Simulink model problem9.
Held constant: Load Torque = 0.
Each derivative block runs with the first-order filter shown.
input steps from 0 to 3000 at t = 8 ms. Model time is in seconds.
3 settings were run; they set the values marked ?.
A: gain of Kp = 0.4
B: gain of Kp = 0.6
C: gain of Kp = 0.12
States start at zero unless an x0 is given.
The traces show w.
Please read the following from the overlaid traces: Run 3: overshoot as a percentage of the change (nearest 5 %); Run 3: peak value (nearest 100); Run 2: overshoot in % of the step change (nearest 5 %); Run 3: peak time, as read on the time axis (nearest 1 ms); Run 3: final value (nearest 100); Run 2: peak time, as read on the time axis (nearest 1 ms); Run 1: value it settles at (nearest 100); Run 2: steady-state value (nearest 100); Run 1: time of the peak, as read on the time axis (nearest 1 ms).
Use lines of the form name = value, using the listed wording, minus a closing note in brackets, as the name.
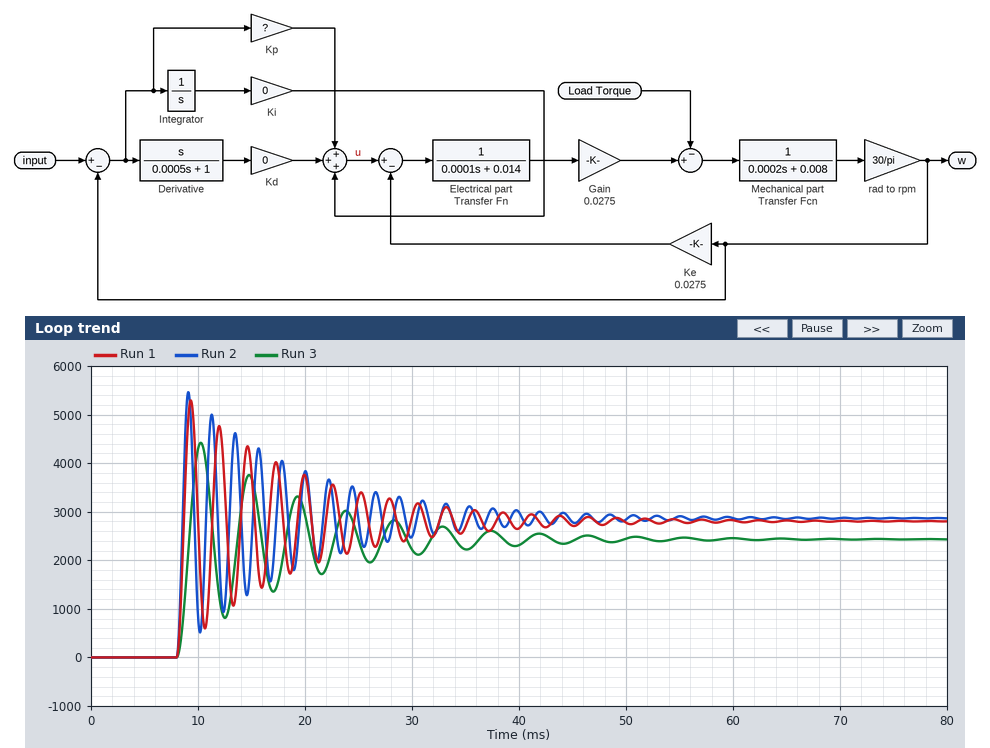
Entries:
Run 3: overshoot as a percentage of the change = 80 %
Run 3: peak value = 4400
Run 2: overshoot in % of the step change = 90 %
Run 3: peak time, as read on the time axis = 10 ms
Run 3: final value = 2400
Run 2: peak time, as read on the time axis = 9 ms
Run 1: value it settles at = 2800
Run 2: steady-state value = 2900
Run 1: time of the peak, as read on the time axis = 9 ms
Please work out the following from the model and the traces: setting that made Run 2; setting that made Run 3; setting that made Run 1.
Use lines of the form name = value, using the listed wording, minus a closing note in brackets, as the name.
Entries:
setting that made Run 2 = B
setting that made Run 3 = C
setting that made Run 1 = A
